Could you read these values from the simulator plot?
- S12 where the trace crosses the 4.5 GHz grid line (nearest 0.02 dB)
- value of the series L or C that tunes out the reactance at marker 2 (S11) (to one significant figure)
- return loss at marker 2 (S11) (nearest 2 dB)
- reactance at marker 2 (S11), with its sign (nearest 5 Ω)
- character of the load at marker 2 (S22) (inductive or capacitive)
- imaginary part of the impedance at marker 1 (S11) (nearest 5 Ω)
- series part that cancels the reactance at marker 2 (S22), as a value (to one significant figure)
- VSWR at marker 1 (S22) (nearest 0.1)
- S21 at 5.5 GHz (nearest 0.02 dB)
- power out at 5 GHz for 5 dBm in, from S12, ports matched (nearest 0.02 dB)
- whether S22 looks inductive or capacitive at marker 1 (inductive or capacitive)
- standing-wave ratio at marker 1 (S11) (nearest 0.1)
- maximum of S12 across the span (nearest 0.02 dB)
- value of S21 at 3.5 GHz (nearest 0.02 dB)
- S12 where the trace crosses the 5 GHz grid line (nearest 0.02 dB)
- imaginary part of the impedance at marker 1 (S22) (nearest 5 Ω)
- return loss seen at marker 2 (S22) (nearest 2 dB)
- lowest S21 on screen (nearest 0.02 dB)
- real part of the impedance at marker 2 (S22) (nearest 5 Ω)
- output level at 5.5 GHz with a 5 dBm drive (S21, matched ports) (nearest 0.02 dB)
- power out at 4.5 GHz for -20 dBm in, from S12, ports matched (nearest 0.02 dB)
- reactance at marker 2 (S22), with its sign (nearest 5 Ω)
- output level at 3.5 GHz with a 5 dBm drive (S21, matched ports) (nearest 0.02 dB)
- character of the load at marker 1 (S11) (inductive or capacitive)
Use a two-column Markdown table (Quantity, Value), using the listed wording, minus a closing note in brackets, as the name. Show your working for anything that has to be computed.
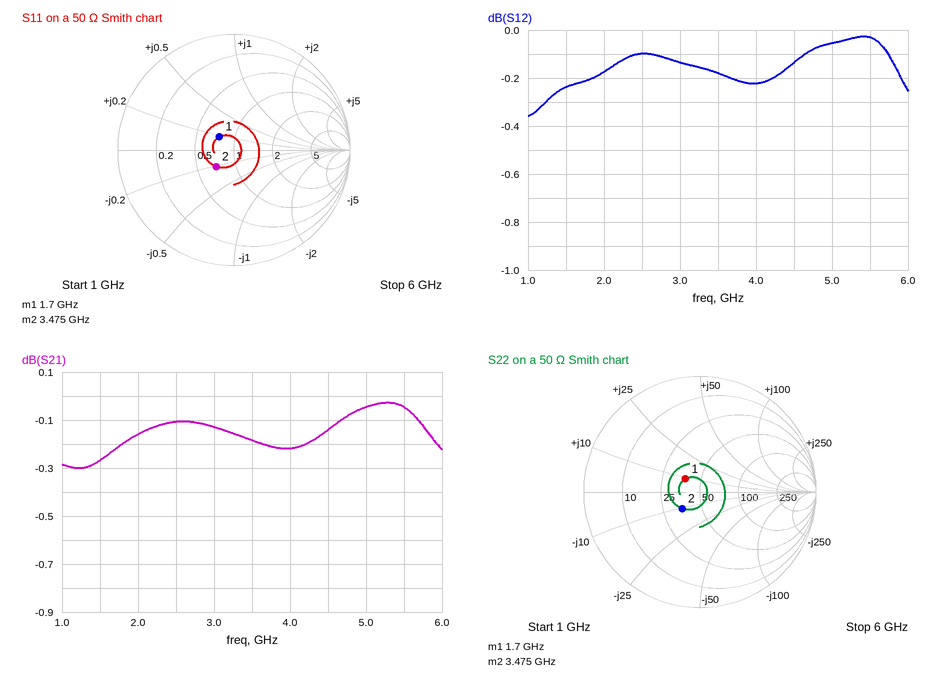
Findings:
| Quantity | Value |
|---|---|
| S12 where the trace crosses the 4.5 GHz grid line | -0.14 dB |
| value of the series L or C that tunes out the reactance at marker 2 (S11) | L = 10 Ω/(2π × 3.475 GHz) ≈ 458 pH, so 500 pH to one significant figure |
| return loss at marker 2 (S11) | 14 dB |
| reactance at marker 2 (S11), with its sign | -10 Ω |
| character of the load at marker 2 (S22) | capacitive |
| imaginary part of the impedance at marker 1 (S11) | +10 Ω |
| series part that cancels the reactance at marker 2 (S22), as a value | L = 10 Ω/(2π × 3.475 GHz) ≈ 458 pH, so 500 pH to one significant figure |
| VSWR at marker 1 (S22) | 1.4 |
| S21 at 5.5 GHz | -0.04 dB |
| power out at 5 GHz for 5 dBm in, from S12, ports matched | 5 dBm + (-0.06 dB) = 4.94 dBm |
| whether S22 looks inductive or capacitive at marker 1 | inductive |
| standing-wave ratio at marker 1 (S11) | 1.4 |
| maximum of S12 across the span | -0.02 dB |
| value of S21 at 3.5 GHz | -0.18 dB |
| S12 where the trace crosses the 5 GHz grid line | -0.06 dB |
| imaginary part of the impedance at marker 1 (S22) | +10 Ω |
| return loss seen at marker 2 (S22) | 14 dB |
| lowest S21 on screen | -0.30 dB |
| real part of the impedance at marker 2 (S22) | 35 Ω |
| output level at 5.5 GHz with a 5 dBm drive (S21, matched ports) | 5 dBm + (-0.04 dB) = 4.96 dBm |
| power out at 4.5 GHz for -20 dBm in, from S12, ports matched | -20 dBm + (-0.14 dB) = -20.14 dBm |
| reactance at marker 2 (S22), with its sign | -10 Ω |
| output level at 3.5 GHz with a 5 dBm drive (S21, matched ports) | 5 dBm + (-0.18 dB) = 4.82 dBm |
| character of the load at marker 1 (S11) | inductive |
